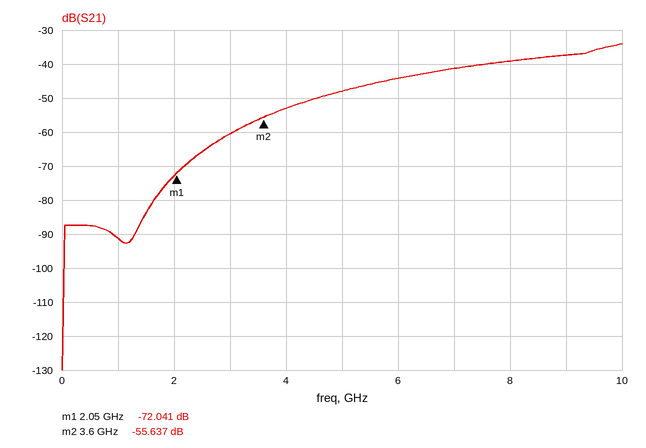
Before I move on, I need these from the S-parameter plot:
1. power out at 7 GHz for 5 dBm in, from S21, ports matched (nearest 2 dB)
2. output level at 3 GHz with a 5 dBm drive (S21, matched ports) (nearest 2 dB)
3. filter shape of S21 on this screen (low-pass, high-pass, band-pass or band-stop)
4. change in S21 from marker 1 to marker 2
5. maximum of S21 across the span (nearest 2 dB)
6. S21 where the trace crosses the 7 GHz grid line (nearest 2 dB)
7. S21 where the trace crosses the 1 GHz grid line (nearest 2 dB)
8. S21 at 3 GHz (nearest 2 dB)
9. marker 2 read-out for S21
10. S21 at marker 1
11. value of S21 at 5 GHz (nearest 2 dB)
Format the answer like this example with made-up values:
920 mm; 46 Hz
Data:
-36 dBm; -56 dBm; high-pass; 16.404 dB; -34 dB; -42 dB; -92 dB; -60 dB; -55.637 dB; -72.041 dB; -48 dB
